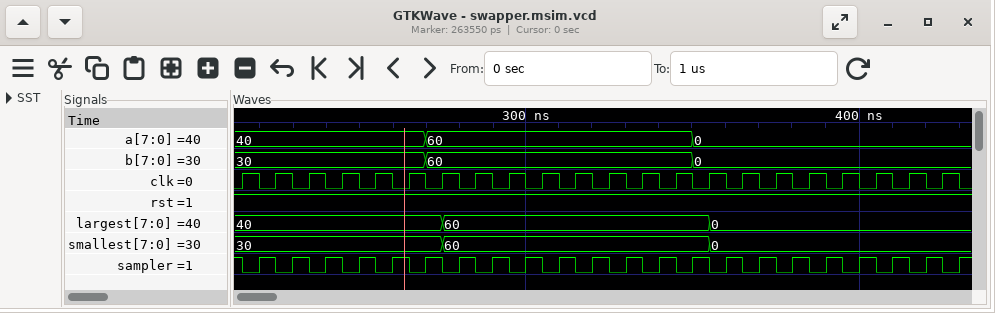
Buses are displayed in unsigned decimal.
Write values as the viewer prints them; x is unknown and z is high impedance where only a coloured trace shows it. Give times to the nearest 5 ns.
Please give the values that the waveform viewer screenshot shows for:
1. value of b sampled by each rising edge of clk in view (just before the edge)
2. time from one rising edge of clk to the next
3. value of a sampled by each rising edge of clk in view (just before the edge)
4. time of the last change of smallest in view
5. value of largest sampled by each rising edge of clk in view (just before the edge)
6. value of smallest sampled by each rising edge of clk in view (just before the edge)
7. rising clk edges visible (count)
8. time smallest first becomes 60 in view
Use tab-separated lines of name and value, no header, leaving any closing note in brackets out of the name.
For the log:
value of b sampled by each rising edge of clk in view	30, 30, 30, 30, 30, 30, 60, 60, 60, 60, 60, 60, 60, 60, 0, 0, 0, 0, 0, 0, 0, 0
time from one rising edge of clk to the next	10 ns
value of a sampled by each rising edge of clk in view	40, 40, 40, 40, 40, 40, 60, 60, 60, 60, 60, 60, 60, 60, 0, 0, 0, 0, 0, 0, 0, 0
time of the last change of smallest in view	355 ns
value of largest sampled by each rising edge of clk in view	40, 40, 40, 40, 40, 40, 40, 60, 60, 60, 60, 60, 60, 60, 60, 0, 0, 0, 0, 0, 0, 0
value of smallest sampled by each rising edge of clk in view	30, 30, 30, 30, 30, 30, 30, 60, 60, 60, 60, 60, 60, 60, 60, 0, 0, 0, 0, 0, 0, 0
rising clk edges visible	22
time smallest first becomes 60 in view	275 ns
